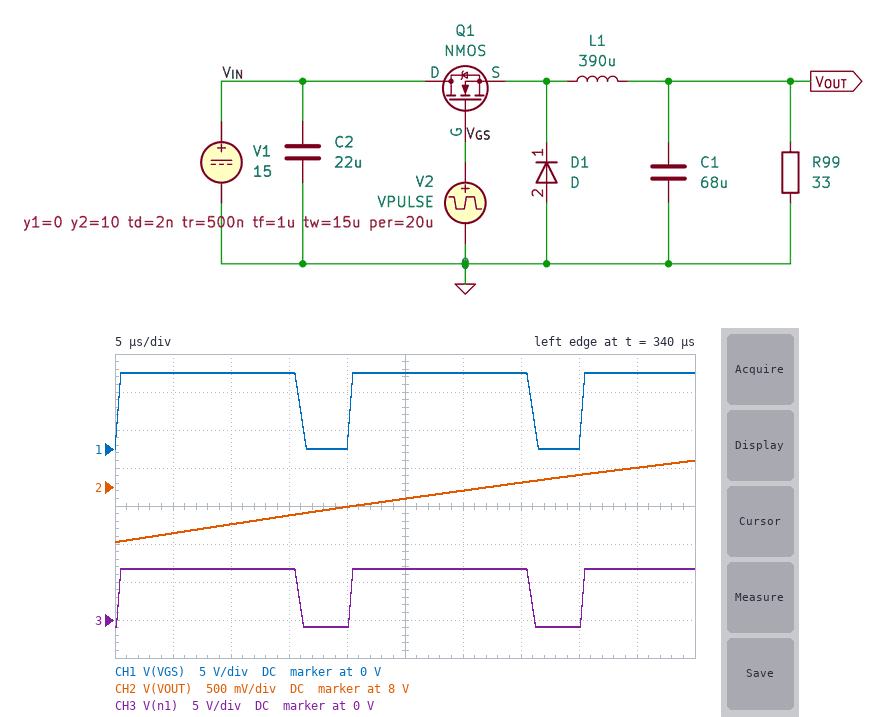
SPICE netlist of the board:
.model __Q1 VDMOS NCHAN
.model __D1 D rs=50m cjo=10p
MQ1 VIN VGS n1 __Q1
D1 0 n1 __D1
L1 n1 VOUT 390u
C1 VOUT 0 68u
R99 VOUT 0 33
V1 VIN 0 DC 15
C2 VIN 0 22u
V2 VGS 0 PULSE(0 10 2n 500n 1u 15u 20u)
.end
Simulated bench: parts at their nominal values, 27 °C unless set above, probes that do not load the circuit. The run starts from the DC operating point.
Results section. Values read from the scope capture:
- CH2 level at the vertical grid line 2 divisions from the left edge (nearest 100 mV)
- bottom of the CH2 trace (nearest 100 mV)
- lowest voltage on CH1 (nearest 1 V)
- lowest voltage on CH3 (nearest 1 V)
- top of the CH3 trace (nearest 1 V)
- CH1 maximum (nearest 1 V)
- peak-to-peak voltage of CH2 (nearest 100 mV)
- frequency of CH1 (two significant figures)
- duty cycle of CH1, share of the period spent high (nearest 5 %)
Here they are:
7.5 V
7.3 V
0 V
-1 V
7 V
10 V
1.1 V
50 kHz
80 %
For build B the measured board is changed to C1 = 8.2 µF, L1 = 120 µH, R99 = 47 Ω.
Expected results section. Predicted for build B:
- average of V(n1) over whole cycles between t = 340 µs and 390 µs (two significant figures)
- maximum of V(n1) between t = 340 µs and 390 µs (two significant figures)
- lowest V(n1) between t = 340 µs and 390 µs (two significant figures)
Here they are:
5.8 V
16 V
-800 mV
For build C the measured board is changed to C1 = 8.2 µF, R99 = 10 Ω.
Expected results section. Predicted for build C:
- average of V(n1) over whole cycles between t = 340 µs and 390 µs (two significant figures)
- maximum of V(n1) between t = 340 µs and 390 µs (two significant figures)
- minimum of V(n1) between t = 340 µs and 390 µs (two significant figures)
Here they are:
5.2 V
6.9 V
-840 mV
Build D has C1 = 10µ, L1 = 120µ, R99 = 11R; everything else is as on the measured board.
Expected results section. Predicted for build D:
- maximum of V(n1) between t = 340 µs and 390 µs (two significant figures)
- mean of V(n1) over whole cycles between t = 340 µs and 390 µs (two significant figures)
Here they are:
6.9 V
5.2 V
